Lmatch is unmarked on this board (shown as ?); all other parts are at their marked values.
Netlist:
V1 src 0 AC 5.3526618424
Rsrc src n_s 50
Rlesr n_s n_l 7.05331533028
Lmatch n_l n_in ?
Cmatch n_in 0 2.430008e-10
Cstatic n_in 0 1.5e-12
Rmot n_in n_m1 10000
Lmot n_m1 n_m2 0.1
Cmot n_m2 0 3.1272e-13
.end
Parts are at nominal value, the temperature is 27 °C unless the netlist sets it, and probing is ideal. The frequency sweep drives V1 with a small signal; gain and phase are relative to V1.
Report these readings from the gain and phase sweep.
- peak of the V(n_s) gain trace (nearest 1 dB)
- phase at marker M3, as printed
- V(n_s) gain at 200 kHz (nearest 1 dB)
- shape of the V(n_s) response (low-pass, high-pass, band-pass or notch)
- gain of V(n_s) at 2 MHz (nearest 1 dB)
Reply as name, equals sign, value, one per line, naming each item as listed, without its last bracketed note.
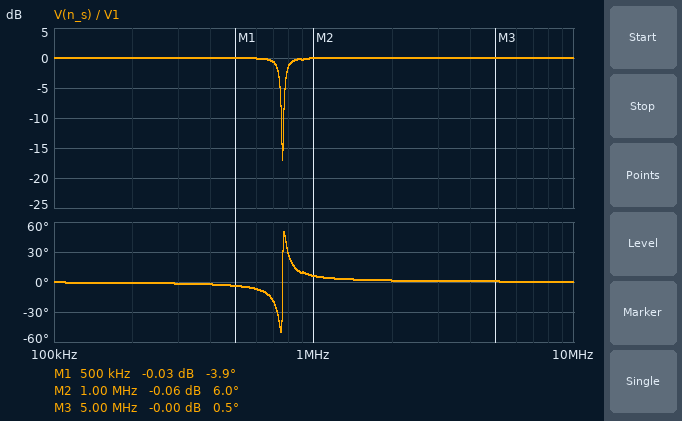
peak of the V(n_s) gain trace = 0 dB
phase at marker M3, as printed = 0.5 deg
V(n_s) gain at 200 kHz = 0 dB
shape of the V(n_s) response = notch
gain of V(n_s) at 2 MHz = 0 dB
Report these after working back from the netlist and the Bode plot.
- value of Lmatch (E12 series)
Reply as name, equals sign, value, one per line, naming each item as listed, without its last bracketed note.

value of Lmatch = 180 µH
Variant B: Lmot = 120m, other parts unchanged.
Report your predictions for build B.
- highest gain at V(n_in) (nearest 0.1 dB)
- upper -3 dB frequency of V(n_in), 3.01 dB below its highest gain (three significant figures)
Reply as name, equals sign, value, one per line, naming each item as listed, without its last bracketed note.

highest gain at V(n_in) = 23.4 dB
upper -3 dB frequency of V(n_in), 3.01 dB below its highest gain = 778 kHz
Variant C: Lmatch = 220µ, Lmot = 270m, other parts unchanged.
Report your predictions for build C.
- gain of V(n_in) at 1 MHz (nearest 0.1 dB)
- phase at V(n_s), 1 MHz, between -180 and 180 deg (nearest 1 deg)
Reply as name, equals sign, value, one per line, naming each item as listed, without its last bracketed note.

gain of V(n_in) at 1 MHz = -1.0 dB
phase at V(n_s), 1 MHz, between -180 and 180 deg = 4 deg
